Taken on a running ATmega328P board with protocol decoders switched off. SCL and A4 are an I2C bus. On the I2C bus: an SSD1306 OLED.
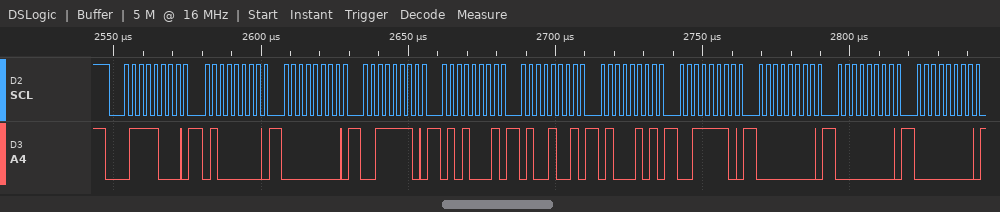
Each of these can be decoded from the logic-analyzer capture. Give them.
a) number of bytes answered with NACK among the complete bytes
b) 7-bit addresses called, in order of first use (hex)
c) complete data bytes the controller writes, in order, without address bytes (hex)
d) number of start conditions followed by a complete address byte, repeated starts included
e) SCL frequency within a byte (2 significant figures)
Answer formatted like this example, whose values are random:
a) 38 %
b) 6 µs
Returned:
a) 0
b) 0x3C
c) 40 00 3E 51 49 45 3E 00 00 00
d) 1
e) 400 kHz
